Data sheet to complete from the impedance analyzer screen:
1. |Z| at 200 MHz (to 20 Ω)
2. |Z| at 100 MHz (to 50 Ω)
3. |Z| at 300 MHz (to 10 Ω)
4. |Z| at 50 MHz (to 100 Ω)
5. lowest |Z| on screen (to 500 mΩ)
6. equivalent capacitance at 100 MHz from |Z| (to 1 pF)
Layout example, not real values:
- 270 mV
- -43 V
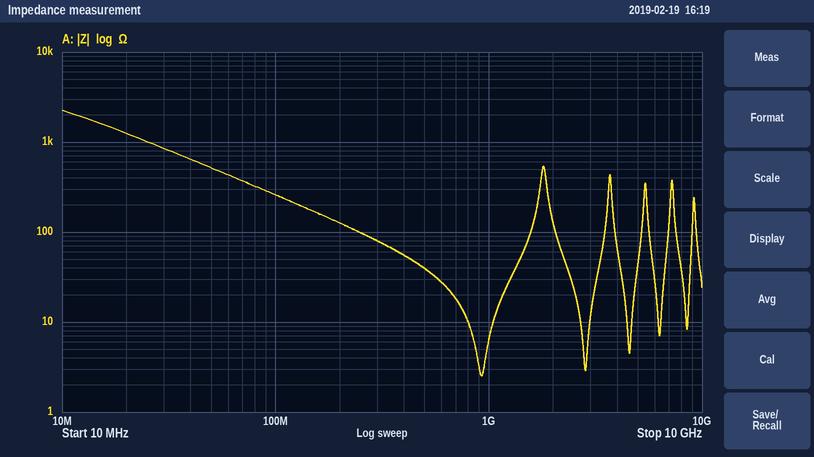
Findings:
- 120 Ω
- 250 Ω
- 80 Ω
- 500 Ω
- 2.5 Ω
- 6 pF
